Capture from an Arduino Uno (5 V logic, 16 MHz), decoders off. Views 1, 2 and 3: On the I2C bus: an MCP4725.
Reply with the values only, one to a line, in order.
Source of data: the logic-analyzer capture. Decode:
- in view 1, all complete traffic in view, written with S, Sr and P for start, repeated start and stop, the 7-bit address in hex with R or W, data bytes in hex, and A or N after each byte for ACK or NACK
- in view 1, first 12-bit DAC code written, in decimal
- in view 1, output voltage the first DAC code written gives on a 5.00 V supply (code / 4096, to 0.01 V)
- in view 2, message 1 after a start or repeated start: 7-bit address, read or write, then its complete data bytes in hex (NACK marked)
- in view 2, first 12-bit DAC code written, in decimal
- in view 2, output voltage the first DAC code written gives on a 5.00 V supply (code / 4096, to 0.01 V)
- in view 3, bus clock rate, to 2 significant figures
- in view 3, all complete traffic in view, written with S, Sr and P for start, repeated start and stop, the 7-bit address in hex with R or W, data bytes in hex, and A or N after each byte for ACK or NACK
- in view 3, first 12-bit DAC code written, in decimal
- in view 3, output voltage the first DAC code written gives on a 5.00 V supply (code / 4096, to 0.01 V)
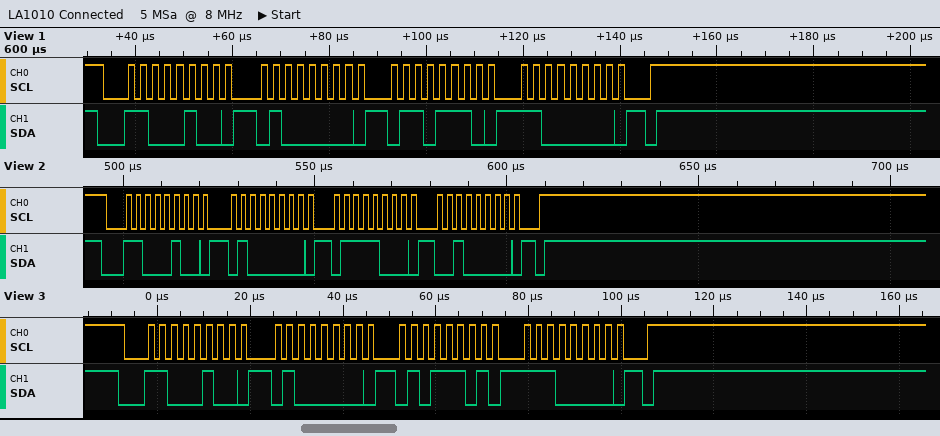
S 62W A 40 A 6E A C0 A P
1772
2.16 V
0x62 write: 40 78 20
1922
2.35 V
400 kHz
S 62W A 40 A 5D A E0 A P
1502
1.83 V
